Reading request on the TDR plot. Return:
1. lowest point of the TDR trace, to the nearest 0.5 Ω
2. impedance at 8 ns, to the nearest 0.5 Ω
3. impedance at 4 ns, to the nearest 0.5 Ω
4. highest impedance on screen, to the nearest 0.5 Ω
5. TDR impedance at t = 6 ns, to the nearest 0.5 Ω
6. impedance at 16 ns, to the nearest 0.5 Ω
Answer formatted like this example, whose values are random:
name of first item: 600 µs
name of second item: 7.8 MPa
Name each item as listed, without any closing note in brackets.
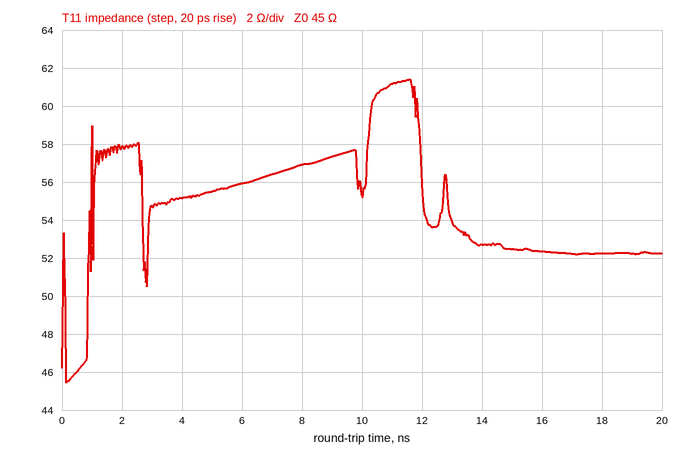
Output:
lowest point of the TDR trace, to the nearest 0.5 Ω: 45.5 Ω
impedance at 8 ns, to the nearest 0.5 Ω: 57.0 Ω
impedance at 4 ns, to the nearest 0.5 Ω: 55.0 Ω
highest impedance on screen, to the nearest 0.5 Ω: 61.5 Ω
TDR impedance at t = 6 ns, to the nearest 0.5 Ω: 56.0 Ω
impedance at 16 ns, to the nearest 0.5 Ω: 52.5 Ω
